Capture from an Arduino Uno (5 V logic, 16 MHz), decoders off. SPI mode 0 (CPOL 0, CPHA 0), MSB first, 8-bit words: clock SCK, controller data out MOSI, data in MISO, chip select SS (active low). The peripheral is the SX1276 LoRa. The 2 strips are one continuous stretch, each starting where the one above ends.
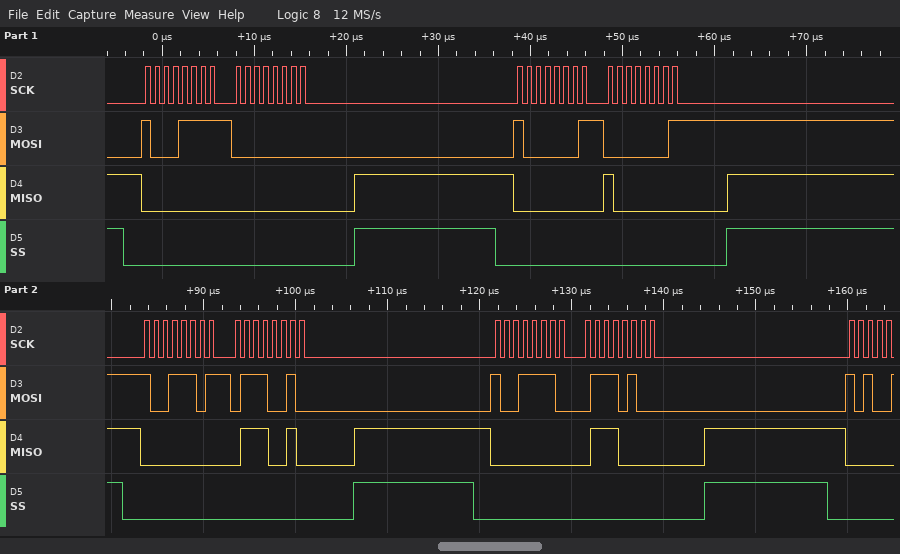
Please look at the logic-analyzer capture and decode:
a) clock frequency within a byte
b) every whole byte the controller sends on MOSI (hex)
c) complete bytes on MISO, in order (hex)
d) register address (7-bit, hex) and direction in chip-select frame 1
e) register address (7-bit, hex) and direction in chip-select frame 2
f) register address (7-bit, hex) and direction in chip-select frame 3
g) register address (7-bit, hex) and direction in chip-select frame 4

1 MHz
0x8F 0x00 0x81 0x01 0x9D 0x72 0x9E 0x74
0x00 0x00 0x00 0x80 0x00 0x72 0x00 0x70
0x0F write
0x01 write
0x1D write
0x1E write
